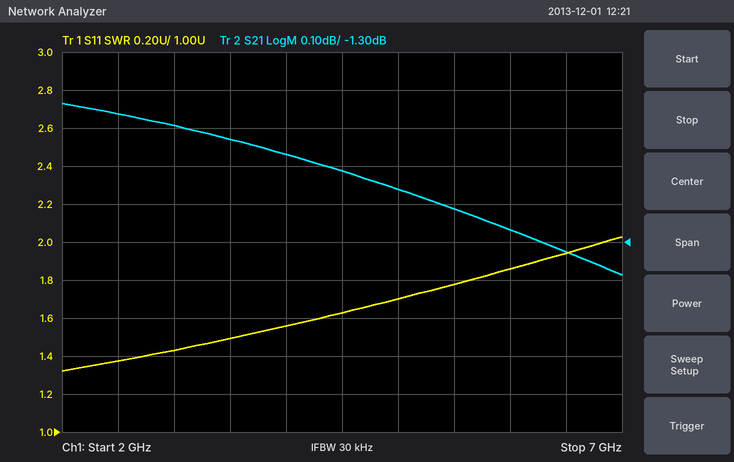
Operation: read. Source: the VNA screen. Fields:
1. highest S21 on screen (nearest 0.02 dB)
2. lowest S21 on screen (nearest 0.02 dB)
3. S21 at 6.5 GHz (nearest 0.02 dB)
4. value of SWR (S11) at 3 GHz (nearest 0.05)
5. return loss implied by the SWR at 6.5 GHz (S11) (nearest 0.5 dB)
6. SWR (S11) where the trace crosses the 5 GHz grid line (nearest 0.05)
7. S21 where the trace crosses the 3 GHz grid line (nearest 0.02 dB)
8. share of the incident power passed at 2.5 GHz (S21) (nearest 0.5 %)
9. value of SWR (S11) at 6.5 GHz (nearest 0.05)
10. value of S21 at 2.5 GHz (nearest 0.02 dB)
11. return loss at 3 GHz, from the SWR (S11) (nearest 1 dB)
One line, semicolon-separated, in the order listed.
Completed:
-0.94 dB; -1.38 dB; -1.32 dB; 1.45; 10.0 dB; 1.70; -1.00 dB; 80.0 %; 1.95; -0.96 dB; 15 dB
